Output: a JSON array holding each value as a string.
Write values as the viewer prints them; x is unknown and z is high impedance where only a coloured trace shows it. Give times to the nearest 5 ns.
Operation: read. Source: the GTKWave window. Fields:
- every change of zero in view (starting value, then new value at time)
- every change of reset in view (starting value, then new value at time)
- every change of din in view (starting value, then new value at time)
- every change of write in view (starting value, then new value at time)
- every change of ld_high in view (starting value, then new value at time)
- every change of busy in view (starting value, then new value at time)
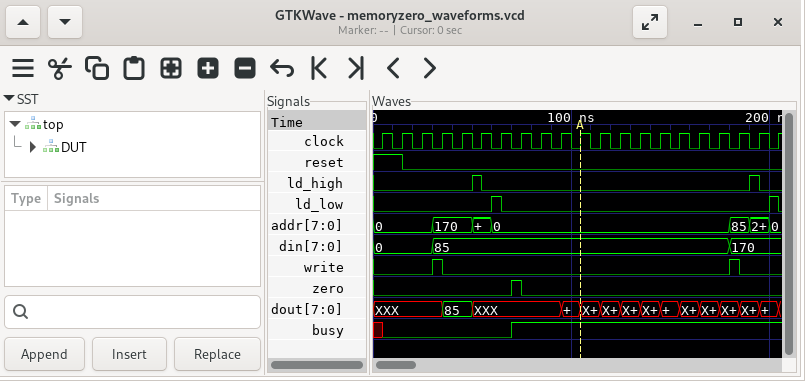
["0, 1 at 70 ns, 0 at 75 ns", "1, 0 at 15 ns", "0, 85 at 30 ns, 170 at 180 ns", "0, 1 at 30 ns, 0 at 35 ns, 1 at 180 ns, 0 at 185 ns", "0, 1 at 50 ns, 0 at 55 ns, 1 at 190 ns, 0 at 195 ns", "x, 0 at 5 ns, 1 at 70 ns"]
